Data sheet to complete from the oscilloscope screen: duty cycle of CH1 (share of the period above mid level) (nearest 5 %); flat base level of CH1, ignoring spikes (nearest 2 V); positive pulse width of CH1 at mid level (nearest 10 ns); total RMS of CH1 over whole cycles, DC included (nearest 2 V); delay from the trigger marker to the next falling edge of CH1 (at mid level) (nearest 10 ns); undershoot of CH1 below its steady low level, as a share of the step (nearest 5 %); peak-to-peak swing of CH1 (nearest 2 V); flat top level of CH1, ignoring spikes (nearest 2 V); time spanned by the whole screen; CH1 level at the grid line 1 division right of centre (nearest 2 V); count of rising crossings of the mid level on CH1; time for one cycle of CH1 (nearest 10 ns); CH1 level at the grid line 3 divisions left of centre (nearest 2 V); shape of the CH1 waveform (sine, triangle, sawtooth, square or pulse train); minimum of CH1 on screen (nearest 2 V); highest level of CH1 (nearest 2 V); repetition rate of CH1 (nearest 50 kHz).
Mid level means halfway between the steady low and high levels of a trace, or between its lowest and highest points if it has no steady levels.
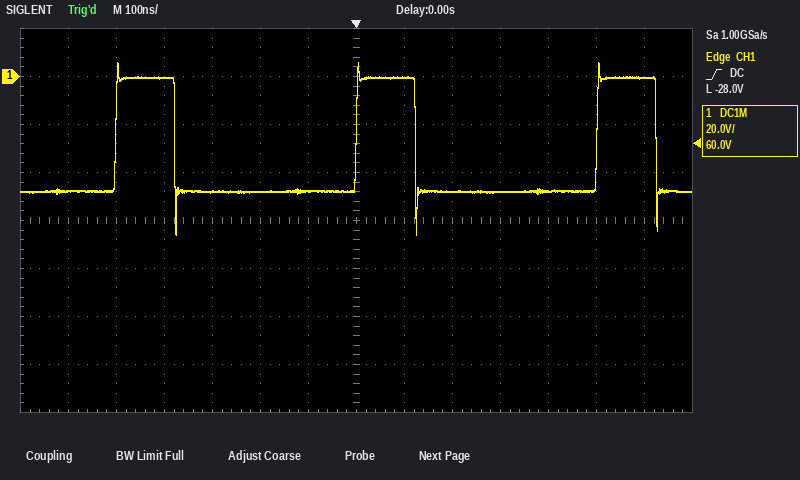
25 %
-48 V
120 ns
42 V
120 ns
40 %
72 V
0 V
1.4 µs
0 V
3
500 ns
-48 V
pulse train
-66 V
6 V
2.00 MHz
